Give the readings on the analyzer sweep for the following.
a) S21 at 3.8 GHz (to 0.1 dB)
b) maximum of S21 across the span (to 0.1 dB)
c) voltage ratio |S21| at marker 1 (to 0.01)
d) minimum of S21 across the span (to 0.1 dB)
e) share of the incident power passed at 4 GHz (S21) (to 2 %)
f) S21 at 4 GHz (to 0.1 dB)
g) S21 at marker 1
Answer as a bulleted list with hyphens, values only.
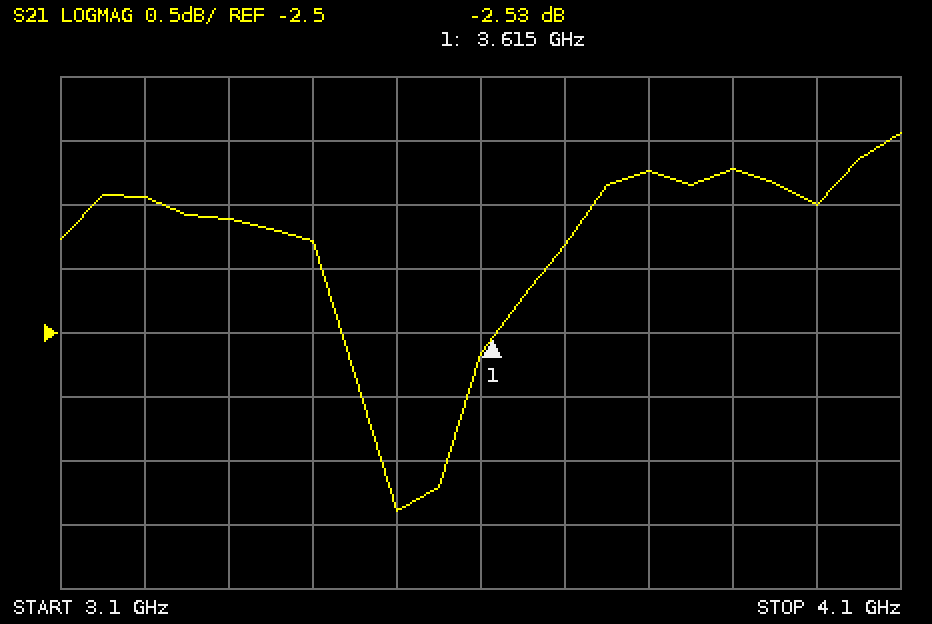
- -1.2 dB
- -0.9 dB
- 0.75
- -3.9 dB
- 70 %
- -1.5 dB
- -2.53 dB
